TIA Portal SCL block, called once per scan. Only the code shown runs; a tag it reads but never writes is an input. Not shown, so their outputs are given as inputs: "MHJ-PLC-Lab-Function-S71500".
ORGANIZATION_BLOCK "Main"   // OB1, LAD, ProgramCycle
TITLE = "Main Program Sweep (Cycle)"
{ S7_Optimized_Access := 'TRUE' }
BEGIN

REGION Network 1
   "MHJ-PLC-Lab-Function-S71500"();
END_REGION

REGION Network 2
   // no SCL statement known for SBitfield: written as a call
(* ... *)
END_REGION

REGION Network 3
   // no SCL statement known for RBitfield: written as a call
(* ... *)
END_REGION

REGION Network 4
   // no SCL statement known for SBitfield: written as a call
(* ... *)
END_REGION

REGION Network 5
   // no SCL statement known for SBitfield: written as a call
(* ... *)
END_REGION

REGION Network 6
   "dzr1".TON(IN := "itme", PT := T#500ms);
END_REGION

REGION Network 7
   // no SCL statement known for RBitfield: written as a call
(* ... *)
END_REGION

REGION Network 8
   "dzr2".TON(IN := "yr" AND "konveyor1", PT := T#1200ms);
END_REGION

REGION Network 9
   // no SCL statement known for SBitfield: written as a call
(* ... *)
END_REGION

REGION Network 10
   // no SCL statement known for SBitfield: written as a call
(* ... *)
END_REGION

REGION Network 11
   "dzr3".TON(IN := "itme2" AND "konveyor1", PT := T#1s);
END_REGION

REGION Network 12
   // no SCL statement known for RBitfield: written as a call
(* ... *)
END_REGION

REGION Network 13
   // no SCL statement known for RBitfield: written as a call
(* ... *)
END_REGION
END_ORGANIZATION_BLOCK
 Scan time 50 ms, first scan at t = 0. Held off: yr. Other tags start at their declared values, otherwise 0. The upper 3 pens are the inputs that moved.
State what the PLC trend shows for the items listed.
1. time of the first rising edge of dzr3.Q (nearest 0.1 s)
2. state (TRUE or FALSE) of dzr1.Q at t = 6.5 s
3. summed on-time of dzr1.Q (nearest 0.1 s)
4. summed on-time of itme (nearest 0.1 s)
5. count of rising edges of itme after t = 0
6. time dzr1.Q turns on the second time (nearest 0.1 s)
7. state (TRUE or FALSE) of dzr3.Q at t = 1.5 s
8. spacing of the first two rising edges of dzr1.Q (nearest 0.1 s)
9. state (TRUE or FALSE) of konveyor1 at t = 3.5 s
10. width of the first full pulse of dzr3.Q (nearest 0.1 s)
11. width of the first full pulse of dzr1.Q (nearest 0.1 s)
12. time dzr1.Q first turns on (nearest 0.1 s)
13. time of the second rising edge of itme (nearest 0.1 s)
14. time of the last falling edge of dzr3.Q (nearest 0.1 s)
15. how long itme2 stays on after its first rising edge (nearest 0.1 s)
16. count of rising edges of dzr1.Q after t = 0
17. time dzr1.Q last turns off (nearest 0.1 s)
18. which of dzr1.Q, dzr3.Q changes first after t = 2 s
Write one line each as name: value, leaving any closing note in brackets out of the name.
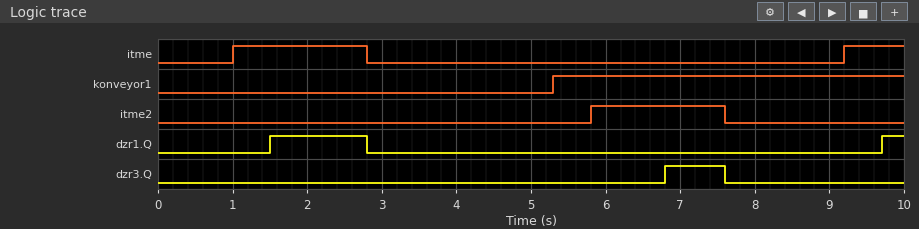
time of the first rising edge of dzr3.Q: 6.8 s
state (TRUE or FALSE) of dzr1.Q at t = 6.5 s: FALSE
summed on-time of dzr1.Q: 1.6 s
summed on-time of itme: 2.6 s
count of rising edges of itme after t = 0: 2
time dzr1.Q turns on the second time: 9.7 s
state (TRUE or FALSE) of dzr3.Q at t = 1.5 s: FALSE
spacing of the first two rising edges of dzr1.Q: 8.2 s
state (TRUE or FALSE) of konveyor1 at t = 3.5 s: FALSE
width of the first full pulse of dzr3.Q: 0.8 s
width of the first full pulse of dzr1.Q: 1.3 s
time dzr1.Q first turns on: 1.5 s
time of the second rising edge of itme: 9.2 s
time of the last falling edge of dzr3.Q: 7.6 s
how long itme2 stays on after its first rising edge: 1.8 s
count of rising edges of dzr1.Q after t = 0: 2
time dzr1.Q last turns off: 2.8 s
which of dzr1.Q, dzr3.Q changes first after t = 2 s: dzr1.Q
